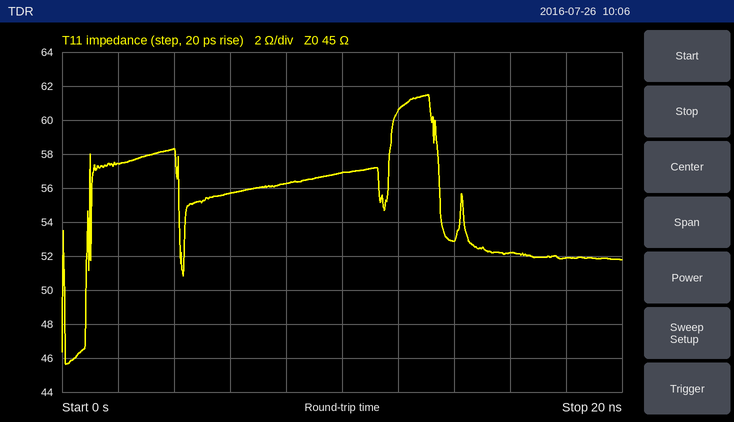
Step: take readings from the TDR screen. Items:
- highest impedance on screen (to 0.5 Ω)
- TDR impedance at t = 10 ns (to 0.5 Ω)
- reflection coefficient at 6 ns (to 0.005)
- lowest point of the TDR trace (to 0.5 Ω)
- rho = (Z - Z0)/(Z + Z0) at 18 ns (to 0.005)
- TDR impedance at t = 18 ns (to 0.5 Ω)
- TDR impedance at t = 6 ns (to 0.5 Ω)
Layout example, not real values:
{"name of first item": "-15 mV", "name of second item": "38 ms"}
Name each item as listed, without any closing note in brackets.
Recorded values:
{"highest impedance on screen": "61.5 Ω", "TDR impedance at t = 10 ns": "57.0 Ω", "reflection coefficient at 6 ns": "+0.105", "lowest point of the TDR trace": "45.5 Ω", "rho = (Z - Z0)/(Z + Z0) at 18 ns": "+0.070", "TDR impedance at t = 18 ns": "52.0 Ω", "TDR impedance at t = 6 ns": "55.5 Ω"}
